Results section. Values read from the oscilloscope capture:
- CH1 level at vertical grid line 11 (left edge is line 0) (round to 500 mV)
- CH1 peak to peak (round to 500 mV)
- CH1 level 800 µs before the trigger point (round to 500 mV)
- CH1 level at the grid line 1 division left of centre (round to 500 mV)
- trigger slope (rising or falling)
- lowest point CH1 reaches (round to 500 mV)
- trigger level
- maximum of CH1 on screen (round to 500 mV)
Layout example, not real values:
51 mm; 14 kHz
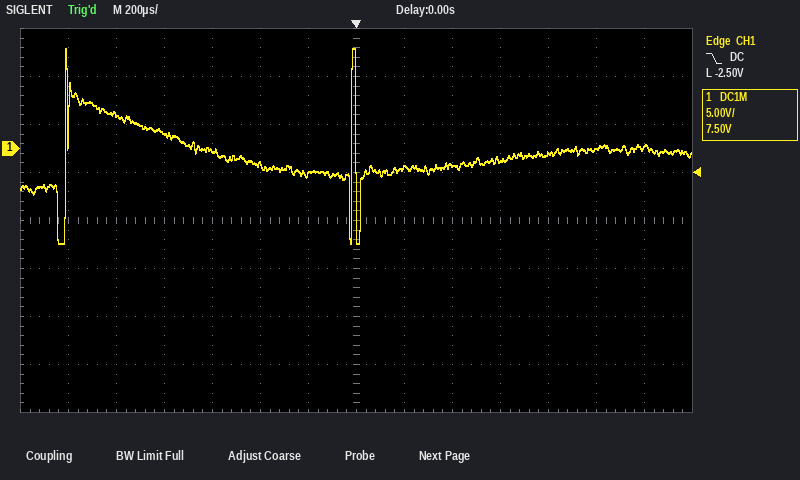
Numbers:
-500 mV; 20.5 V; 1.5 V; -2.5 V; falling; -10.0 V; -2.50 V; 10.5 V
